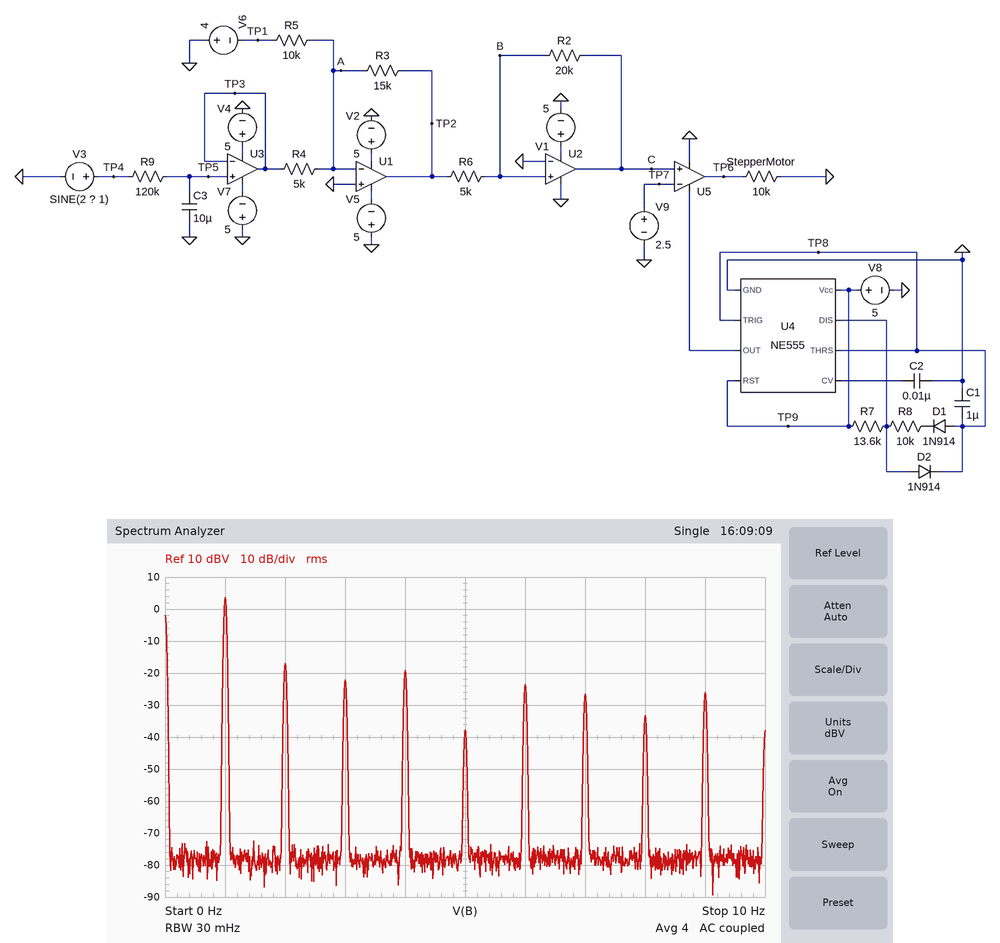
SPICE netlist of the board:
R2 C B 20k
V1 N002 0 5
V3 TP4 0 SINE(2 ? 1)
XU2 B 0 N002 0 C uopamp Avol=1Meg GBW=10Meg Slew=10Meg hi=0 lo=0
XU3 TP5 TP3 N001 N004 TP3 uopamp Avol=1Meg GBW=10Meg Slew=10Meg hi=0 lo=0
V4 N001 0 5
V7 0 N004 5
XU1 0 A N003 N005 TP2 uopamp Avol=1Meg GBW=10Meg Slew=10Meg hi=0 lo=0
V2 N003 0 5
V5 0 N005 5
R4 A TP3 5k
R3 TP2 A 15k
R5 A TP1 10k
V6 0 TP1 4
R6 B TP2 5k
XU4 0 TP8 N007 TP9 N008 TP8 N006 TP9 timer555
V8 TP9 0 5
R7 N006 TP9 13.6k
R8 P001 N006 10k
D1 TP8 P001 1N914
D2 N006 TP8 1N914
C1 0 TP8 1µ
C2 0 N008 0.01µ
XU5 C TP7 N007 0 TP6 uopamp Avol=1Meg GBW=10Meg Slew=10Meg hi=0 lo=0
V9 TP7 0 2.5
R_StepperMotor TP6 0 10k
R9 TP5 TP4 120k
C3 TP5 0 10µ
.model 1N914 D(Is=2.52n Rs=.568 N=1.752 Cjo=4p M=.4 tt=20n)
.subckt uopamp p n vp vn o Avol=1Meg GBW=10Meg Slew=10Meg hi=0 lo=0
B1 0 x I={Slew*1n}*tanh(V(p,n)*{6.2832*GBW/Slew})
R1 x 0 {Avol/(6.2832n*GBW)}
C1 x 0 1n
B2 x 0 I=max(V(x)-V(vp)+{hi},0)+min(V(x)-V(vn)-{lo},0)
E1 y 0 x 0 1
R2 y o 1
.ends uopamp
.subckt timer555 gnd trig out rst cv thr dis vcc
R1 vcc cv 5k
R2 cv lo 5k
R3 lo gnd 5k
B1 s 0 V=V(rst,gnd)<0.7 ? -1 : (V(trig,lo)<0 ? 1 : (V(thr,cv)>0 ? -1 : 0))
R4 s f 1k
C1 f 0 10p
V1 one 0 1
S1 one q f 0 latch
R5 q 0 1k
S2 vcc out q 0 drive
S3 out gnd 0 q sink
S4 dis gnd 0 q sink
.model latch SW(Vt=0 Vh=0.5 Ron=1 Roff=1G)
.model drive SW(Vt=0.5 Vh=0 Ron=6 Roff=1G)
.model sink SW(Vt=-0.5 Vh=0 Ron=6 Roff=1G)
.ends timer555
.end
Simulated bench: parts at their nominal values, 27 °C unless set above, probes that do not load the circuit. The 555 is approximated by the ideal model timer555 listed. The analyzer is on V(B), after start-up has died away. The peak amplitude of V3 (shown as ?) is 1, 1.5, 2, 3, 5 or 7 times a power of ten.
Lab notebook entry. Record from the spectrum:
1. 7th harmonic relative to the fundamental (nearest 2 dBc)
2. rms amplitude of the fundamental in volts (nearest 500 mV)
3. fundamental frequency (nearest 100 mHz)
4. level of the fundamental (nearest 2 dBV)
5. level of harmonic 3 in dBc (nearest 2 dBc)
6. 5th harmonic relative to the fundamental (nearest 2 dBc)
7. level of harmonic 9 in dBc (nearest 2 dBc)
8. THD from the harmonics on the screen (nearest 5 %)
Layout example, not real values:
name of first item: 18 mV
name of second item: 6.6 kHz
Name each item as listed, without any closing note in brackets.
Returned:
7th harmonic relative to the fundamental: -30 dBc
rms amplitude of the fundamental in volts: 1.5 V
fundamental frequency: 1.0 Hz
level of the fundamental: 4 dBV
level of harmonic 3 in dBc: -26 dBc
5th harmonic relative to the fundamental: -42 dBc
level of harmonic 9 in dBc: -30 dBc
THD from the harmonics on the screen: 15 %
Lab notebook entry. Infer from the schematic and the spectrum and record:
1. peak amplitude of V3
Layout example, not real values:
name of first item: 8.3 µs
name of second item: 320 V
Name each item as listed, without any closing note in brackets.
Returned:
peak amplitude of V3: 5 V
